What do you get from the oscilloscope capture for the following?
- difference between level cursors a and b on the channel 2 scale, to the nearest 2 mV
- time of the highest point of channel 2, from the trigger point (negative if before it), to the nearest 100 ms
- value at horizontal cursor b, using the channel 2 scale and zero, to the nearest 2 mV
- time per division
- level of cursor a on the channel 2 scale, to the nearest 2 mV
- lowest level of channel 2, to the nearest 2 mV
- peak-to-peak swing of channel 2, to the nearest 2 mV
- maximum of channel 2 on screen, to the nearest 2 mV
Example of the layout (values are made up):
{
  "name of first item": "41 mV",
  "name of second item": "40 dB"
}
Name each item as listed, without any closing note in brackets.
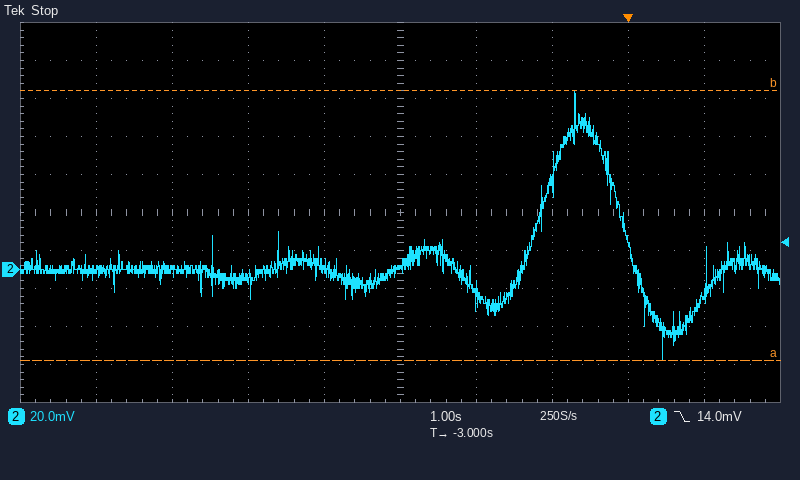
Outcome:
{
  "difference between level cursors a and b on the channel 2 scale, to the nearest 2 mV": "142 mV",
  "time of the highest point of channel 2, from the trigger point (negative if before it), to the nearest 100 ms": "-700 ms",
  "value at horizontal cursor b, using the channel 2 scale and zero, to the nearest 2 mV": "94 mV",
  "time per division": "1 s",
  "level of cursor a on the channel 2 scale, to the nearest 2 mV": "-48 mV",
  "lowest level of channel 2, to the nearest 2 mV": "-48 mV",
  "peak-to-peak swing of channel 2, to the nearest 2 mV": "142 mV",
  "maximum of channel 2 on screen, to the nearest 2 mV": "94 mV"
}
